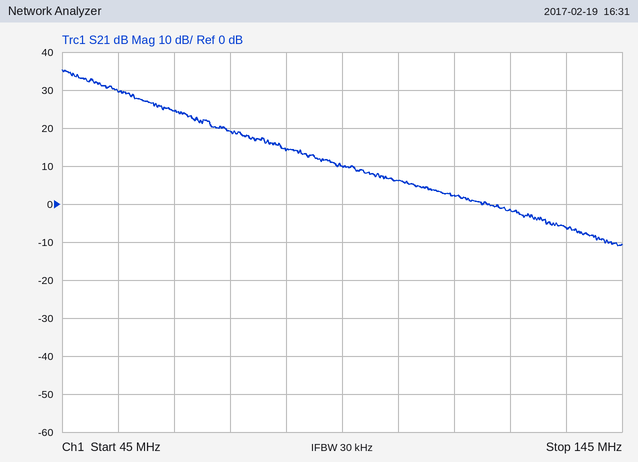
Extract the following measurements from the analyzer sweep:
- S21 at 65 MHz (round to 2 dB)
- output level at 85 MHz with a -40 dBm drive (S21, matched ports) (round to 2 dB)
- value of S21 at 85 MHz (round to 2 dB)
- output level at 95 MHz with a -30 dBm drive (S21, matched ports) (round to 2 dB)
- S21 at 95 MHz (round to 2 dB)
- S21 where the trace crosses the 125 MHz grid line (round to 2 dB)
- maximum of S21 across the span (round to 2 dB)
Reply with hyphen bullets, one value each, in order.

- 24 dB
- -26 dBm
- 14 dB
- -20 dBm
- 10 dB
- -2 dB
- 36 dB
